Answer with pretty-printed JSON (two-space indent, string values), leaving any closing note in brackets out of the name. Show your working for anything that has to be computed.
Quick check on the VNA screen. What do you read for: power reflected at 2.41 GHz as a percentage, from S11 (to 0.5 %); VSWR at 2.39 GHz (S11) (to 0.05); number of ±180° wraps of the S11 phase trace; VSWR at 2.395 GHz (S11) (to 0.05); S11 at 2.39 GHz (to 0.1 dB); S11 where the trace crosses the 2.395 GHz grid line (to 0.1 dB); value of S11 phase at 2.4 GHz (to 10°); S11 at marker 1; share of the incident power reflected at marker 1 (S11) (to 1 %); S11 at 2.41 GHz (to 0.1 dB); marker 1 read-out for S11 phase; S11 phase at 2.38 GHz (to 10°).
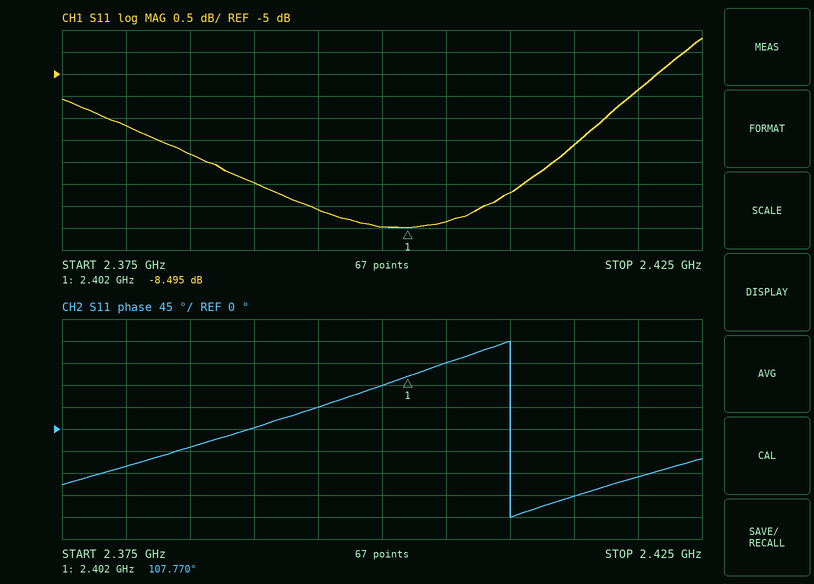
{
  "power reflected at 2.41 GHz as a percentage, from S11": "10^(-7.7/10) ≈ 17.0 %",
  "VSWR at 2.39 GHz (S11)": "|Γ| = 10^(-7.5/20) = 0.4217; VSWR = (1 + 0.4217)/(1 − 0.4217) ≈ 2.46, so 2.45 to the nearest 0.05",
  "number of ±180° wraps of the S11 phase trace": "1",
  "VSWR at 2.395 GHz (S11)": "|Γ| = 10^(-8.1/20) = 0.3936; VSWR = (1 + 0.3936)/(1 − 0.3936) ≈ 2.30",
  "S11 at 2.39 GHz": "-7.5 dB",
  "S11 where the trace crosses the 2.395 GHz grid line": "-8.1 dB",
  "value of S11 phase at 2.4 GHz": "90°",
  "S11 at marker 1": "-8.495 dB",
  "share of the incident power reflected at marker 1 (S11)": "10^(-8.495/10) ≈ 14 %",
  "S11 at 2.41 GHz": "-7.7 dB",
  "marker 1 read-out for S11 phase": "107.770°",
  "S11 phase at 2.38 GHz": "-80°"
}
